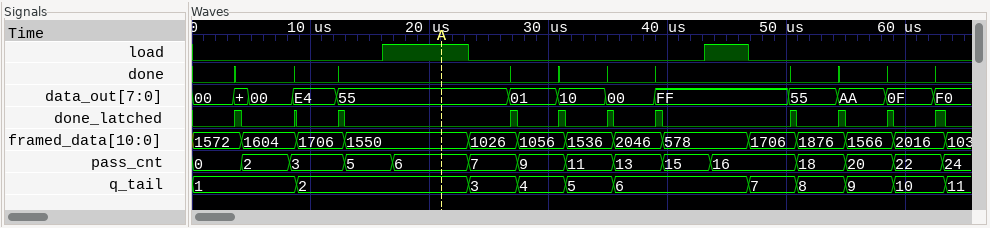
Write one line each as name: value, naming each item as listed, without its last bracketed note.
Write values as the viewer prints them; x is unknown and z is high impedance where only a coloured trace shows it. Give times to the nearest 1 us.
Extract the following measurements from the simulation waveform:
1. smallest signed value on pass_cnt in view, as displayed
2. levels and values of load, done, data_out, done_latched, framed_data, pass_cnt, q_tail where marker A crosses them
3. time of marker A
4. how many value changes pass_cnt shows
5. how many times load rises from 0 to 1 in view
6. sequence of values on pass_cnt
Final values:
smallest signed value on pass_cnt in view, as displayed: 0
levels and values of load, done, data_out, done_latched, framed_data, pass_cnt, q_tail where marker A crosses them: load=1, done=0, data_out=55, done_latched=0, framed_data=1550, pass_cnt=6, q_tail=2
time of marker A: 21 us
how many value changes pass_cnt shows: 14
how many times load rises from 0 to 1 in view: 2
sequence of values on pass_cnt: 0, 2, 3, 5, 6, 7, 9, 11, 13, 15, 16, 18, 20, 22, 24
